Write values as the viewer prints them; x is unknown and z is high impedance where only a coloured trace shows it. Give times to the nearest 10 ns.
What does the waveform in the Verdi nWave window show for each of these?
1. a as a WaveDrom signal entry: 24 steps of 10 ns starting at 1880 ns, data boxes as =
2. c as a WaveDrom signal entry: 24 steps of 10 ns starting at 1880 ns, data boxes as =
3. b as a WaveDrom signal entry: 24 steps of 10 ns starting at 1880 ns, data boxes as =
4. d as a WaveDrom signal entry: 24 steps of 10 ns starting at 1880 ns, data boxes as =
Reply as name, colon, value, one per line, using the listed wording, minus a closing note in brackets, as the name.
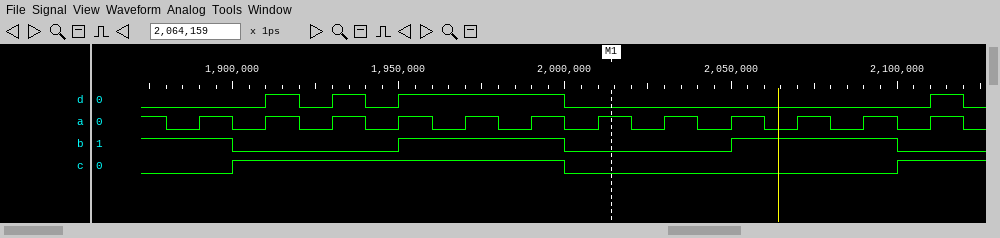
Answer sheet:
a as a WaveDrom signal entry: 24 steps of 10 ns starting at 1880 ns, data boxes as =: {name: 'a', wave: '010101010101010101010101'}
c as a WaveDrom signal entry: 24 steps of 10 ns starting at 1880 ns, data boxes as =: {name: 'c', wave: '0.1.........0.........1.'}
b as a WaveDrom signal entry: 24 steps of 10 ns starting at 1880 ns, data boxes as =: {name: 'b', wave: '1.0....1....0....1....0.'}
d as a WaveDrom signal entry: 24 steps of 10 ns starting at 1880 ns, data boxes as =: {name: 'd', wave: '0..10101....0..........1'}
